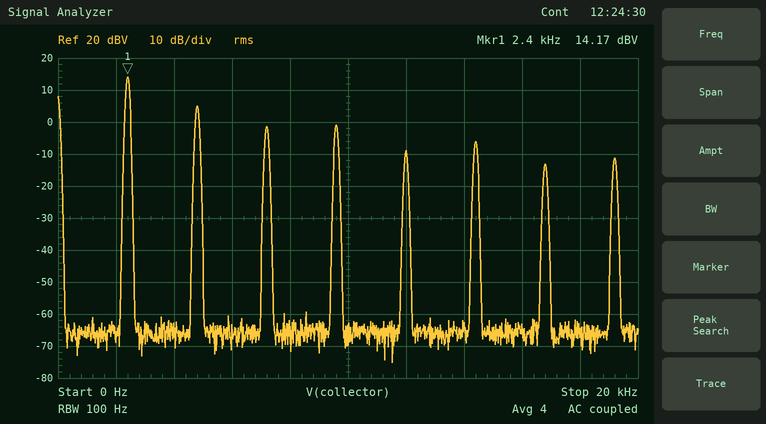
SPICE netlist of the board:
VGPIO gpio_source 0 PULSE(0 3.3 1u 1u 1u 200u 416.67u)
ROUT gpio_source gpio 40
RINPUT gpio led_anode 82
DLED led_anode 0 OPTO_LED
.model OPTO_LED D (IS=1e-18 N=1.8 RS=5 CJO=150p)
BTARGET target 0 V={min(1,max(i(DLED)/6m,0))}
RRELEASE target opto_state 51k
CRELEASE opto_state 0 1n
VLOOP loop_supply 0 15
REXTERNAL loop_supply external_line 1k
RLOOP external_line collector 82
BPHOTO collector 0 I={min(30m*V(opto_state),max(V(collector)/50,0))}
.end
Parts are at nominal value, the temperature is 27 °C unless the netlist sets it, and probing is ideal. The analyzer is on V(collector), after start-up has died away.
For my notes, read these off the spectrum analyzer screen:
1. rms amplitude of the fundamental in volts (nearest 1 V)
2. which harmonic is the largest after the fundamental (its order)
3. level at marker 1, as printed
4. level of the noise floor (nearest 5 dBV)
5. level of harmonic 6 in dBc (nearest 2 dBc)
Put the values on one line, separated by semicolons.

5 V; 2; 14.17 dBV; -65 dBV; -20 dBc
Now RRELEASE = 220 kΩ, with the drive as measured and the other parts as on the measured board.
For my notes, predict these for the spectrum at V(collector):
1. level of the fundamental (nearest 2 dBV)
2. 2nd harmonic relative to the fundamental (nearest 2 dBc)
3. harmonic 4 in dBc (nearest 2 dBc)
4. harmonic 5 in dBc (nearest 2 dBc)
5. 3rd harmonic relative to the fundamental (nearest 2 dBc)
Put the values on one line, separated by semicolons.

4 dBV; -4 dBc; -20 dBc; -20 dBc; -12 dBc
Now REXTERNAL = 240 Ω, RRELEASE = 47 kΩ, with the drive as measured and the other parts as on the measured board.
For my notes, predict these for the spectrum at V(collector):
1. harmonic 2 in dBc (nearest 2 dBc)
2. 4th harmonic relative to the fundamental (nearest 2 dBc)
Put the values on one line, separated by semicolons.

-28 dBc; -32 dBc
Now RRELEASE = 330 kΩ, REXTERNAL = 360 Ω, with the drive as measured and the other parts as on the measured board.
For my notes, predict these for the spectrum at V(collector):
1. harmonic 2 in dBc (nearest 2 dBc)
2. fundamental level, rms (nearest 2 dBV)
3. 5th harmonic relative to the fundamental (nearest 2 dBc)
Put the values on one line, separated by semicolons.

-30 dBc; 2 dBV; -28 dBc
